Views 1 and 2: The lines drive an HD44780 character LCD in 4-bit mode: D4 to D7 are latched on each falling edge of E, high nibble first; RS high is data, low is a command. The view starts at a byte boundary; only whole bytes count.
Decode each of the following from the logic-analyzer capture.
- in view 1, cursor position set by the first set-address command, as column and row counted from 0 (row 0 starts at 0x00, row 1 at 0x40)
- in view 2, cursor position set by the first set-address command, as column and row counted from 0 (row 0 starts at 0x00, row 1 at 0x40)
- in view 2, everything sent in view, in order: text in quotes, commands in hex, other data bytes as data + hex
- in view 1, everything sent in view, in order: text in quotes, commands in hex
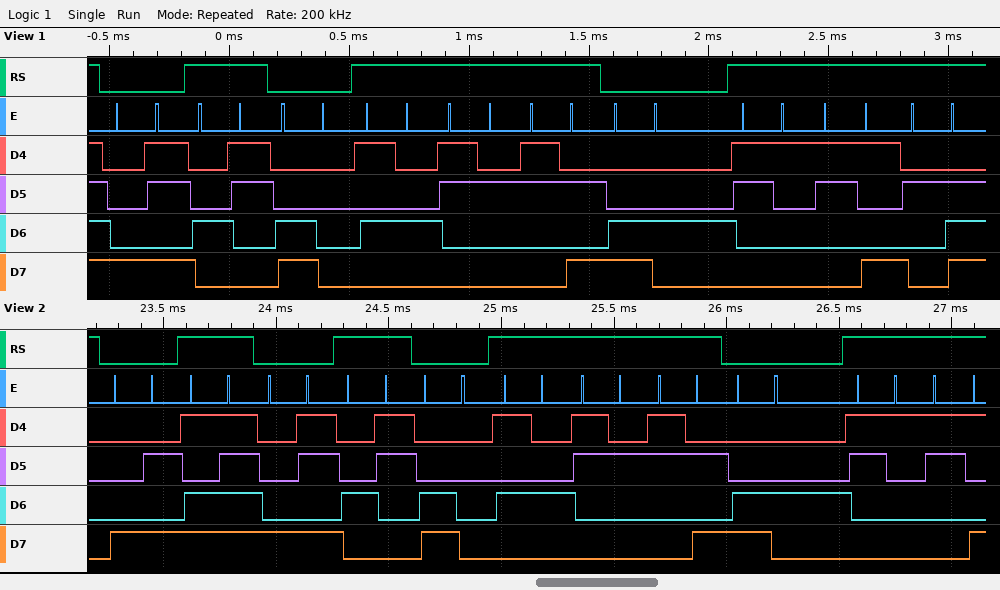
column 11, row 0
column 10, row 0
0x8A data DF 0x8B "C" 0xC0 "T2:" 0xC4 "19"
0x8B "C" 0xC0 "T2:" 0xC4 "19."
